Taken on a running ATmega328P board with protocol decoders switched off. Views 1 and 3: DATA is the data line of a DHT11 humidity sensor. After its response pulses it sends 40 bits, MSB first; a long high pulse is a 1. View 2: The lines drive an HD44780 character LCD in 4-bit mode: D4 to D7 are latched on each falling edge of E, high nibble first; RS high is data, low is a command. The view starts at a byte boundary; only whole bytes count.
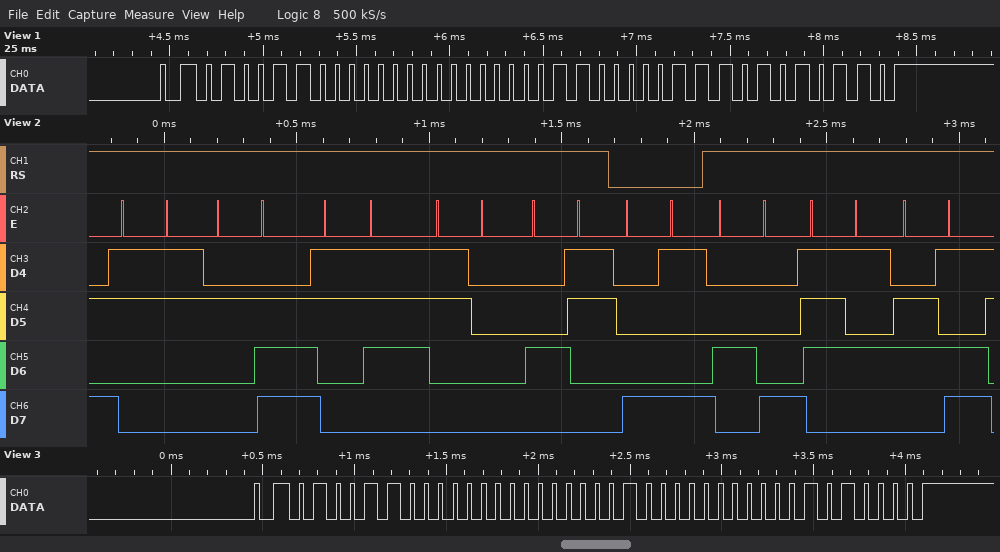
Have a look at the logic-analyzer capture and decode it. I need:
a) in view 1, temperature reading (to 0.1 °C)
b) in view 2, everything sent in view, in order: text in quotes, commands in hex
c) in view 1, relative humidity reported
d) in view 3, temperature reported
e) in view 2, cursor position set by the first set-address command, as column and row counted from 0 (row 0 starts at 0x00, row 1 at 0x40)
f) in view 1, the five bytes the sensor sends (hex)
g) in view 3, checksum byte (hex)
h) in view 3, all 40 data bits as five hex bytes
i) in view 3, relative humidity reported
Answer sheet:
3.7 °C
"3.70C" 0x89 "Hum"
76 %
4.0 °C
column 9, row 0
4C 00 03 07 56
0x50
4C 00 04 00 50
76 %
